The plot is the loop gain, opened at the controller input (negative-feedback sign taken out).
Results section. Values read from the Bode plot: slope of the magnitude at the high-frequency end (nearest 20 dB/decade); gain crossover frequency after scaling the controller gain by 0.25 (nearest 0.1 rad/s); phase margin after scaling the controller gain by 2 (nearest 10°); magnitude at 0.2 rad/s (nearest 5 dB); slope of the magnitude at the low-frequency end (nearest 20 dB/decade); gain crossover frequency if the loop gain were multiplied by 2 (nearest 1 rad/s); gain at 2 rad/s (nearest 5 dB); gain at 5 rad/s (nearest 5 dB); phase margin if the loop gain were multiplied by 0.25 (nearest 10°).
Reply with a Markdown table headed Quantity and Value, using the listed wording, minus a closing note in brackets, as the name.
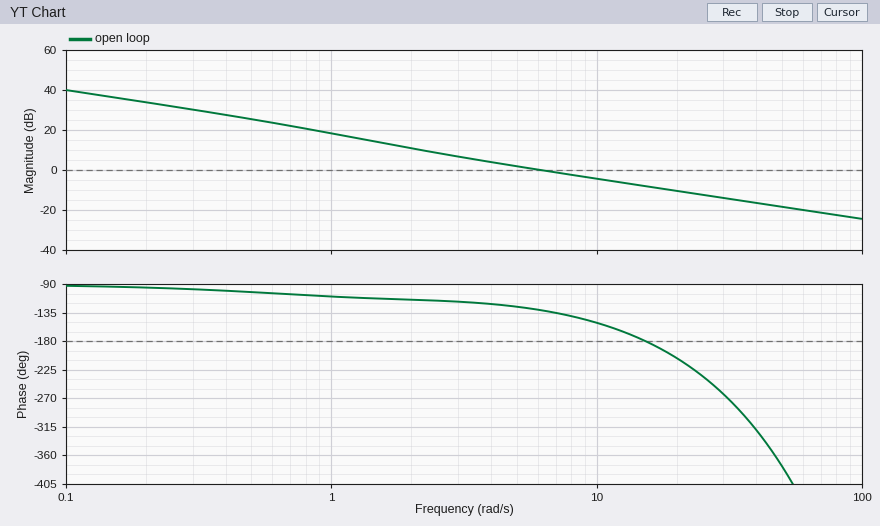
| Quantity | Value |
|---|---|
| slope of the magnitude at the high-frequency end | -20 dB/decade |
| gain crossover frequency after scaling the controller gain by 0.25 | 1.8 rad/s |
| phase margin after scaling the controller gain by 2 | 20° |
| magnitude at 0.2 rad/s | 35 dB |
| slope of the magnitude at the low-frequency end | -20 dB/decade |
| gain crossover frequency if the loop gain were multiplied by 2 | 12 rad/s |
| gain at 2 rad/s | 10 dB |
| gain at 5 rad/s | 0 dB |
| phase margin if the loop gain were multiplied by 0.25 | 70° |
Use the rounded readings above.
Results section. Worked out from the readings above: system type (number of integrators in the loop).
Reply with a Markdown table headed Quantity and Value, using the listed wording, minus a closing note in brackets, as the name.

| Quantity | Value |
|---|---|
| system type | 1 |
